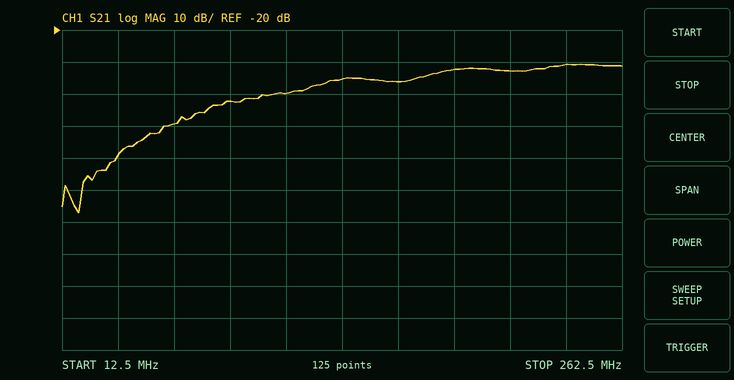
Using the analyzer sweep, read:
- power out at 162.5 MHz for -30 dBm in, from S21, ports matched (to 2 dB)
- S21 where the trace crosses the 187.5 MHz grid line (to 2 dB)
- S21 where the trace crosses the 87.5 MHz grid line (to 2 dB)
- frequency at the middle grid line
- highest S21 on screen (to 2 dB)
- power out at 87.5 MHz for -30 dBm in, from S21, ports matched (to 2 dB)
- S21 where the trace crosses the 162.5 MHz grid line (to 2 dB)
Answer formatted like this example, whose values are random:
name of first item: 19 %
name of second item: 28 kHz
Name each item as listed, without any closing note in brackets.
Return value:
power out at 162.5 MHz for -30 dBm in, from S21, ports matched: -66 dBm
S21 where the trace crosses the 187.5 MHz grid line: -32 dB
S21 where the trace crosses the 87.5 MHz grid line: -42 dB
frequency at the middle grid line: 137.5 MHz
highest S21 on screen: -30 dB
power out at 87.5 MHz for -30 dBm in, from S21, ports matched: -72 dBm
S21 where the trace crosses the 162.5 MHz grid line: -36 dB
